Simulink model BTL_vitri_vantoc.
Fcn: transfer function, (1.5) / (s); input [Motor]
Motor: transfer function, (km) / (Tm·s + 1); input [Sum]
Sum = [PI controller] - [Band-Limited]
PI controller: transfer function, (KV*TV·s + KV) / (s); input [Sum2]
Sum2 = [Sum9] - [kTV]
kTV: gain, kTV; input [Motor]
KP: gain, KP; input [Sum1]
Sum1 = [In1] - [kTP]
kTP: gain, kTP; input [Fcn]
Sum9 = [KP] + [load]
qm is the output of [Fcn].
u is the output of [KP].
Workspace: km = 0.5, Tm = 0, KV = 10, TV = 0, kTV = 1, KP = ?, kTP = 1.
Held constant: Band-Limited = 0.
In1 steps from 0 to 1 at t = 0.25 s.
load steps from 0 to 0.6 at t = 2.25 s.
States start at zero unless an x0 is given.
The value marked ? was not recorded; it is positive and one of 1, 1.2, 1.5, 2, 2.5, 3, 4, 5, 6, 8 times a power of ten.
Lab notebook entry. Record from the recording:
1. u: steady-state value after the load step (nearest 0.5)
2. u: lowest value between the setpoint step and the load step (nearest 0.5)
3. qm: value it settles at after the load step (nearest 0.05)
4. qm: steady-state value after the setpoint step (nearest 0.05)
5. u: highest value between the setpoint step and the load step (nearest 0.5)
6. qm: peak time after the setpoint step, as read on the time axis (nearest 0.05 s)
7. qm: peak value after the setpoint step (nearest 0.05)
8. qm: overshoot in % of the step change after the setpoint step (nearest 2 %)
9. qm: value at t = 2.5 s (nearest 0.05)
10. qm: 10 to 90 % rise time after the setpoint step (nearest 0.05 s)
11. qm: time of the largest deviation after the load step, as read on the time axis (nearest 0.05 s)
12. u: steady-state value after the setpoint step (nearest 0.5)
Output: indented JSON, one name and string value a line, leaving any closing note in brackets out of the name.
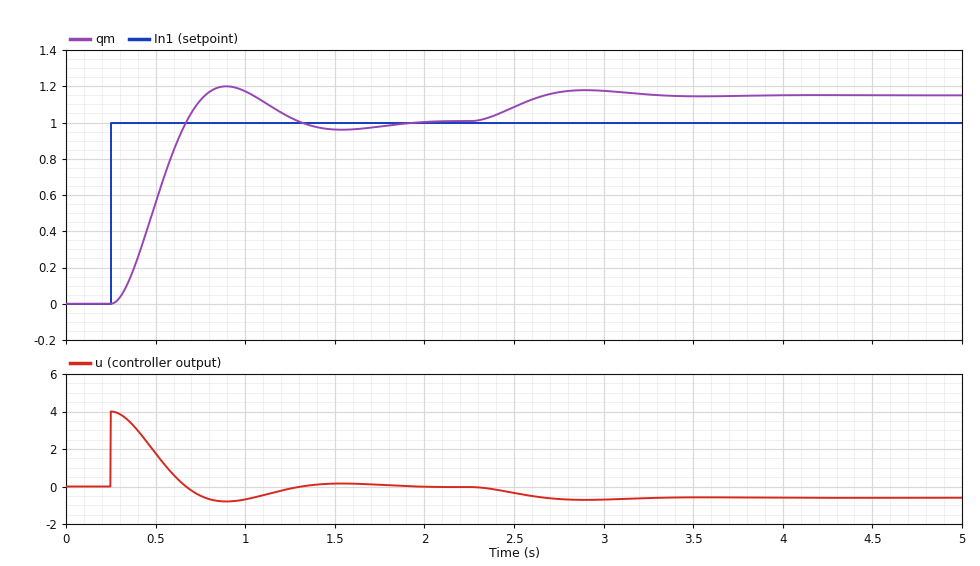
{
  "u: steady-state value after the load step": "-0.5",
  "u: lowest value between the setpoint step and the load step": "-1.0",
  "qm: value it settles at after the load step": "1.15",
  "qm: steady-state value after the setpoint step": "1.00",
  "u: highest value between the setpoint step and the load step": "4.0",
  "qm: peak time after the setpoint step, as read on the time axis": "0.90 s",
  "qm: peak value after the setpoint step": "1.20",
  "qm: overshoot in % of the step change after the setpoint step": "20 %",
  "qm: value at t = 2.5 s": "1.10",
  "qm: 10 to 90 % rise time after the setpoint step": "0.30 s",
  "qm: time of the largest deviation after the load step, as read on the time axis": "2.90 s",
  "u: steady-state value after the setpoint step": "0.0"
}
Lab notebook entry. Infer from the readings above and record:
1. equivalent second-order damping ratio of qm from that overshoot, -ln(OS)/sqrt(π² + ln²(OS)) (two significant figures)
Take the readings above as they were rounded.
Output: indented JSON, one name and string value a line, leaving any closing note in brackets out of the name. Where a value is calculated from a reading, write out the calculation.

{
  "equivalent second-order damping ratio of qm from that overshoot, -ln(OS)/sqrt(π² + ln²(OS))": "ln(0.2) = -1.609; 1.609 / sqrt(9.870 + 2.590) = 0.46"
}
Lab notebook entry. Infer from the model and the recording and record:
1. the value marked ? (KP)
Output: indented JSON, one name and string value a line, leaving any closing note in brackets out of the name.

{
  "the value marked ?": "4"
}
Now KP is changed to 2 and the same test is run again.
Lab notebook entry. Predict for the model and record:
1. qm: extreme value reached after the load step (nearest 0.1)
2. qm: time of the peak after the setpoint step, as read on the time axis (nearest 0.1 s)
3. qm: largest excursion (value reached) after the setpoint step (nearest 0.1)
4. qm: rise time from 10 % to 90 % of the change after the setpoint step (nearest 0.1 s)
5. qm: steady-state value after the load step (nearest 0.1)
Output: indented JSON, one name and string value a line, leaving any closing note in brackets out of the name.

{
  "qm: extreme value reached after the load step": "1.3",
  "qm: time of the peak after the setpoint step, as read on the time axis": "1.3 s",
  "qm: largest excursion (value reached) after the setpoint step": "1.1",
  "qm: rise time from 10 % to 90 % of the change after the setpoint step": "0.5 s",
  "qm: steady-state value after the load step": "1.3"
}
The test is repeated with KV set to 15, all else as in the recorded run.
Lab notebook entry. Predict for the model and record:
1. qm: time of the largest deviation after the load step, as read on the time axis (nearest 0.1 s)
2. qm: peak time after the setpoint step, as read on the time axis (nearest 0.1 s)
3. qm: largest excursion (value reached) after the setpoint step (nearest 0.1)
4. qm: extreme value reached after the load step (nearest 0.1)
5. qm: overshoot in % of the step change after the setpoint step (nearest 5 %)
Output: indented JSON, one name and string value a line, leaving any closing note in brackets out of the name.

{
  "qm: time of the largest deviation after the load step, as read on the time axis": "2.8 s",
  "qm: peak time after the setpoint step, as read on the time axis": "0.8 s",
  "qm: largest excursion (value reached) after the setpoint step": "1.1",
  "qm: extreme value reached after the load step": "1.2",
  "qm: overshoot in % of the step change after the setpoint step": "10 %"
}
